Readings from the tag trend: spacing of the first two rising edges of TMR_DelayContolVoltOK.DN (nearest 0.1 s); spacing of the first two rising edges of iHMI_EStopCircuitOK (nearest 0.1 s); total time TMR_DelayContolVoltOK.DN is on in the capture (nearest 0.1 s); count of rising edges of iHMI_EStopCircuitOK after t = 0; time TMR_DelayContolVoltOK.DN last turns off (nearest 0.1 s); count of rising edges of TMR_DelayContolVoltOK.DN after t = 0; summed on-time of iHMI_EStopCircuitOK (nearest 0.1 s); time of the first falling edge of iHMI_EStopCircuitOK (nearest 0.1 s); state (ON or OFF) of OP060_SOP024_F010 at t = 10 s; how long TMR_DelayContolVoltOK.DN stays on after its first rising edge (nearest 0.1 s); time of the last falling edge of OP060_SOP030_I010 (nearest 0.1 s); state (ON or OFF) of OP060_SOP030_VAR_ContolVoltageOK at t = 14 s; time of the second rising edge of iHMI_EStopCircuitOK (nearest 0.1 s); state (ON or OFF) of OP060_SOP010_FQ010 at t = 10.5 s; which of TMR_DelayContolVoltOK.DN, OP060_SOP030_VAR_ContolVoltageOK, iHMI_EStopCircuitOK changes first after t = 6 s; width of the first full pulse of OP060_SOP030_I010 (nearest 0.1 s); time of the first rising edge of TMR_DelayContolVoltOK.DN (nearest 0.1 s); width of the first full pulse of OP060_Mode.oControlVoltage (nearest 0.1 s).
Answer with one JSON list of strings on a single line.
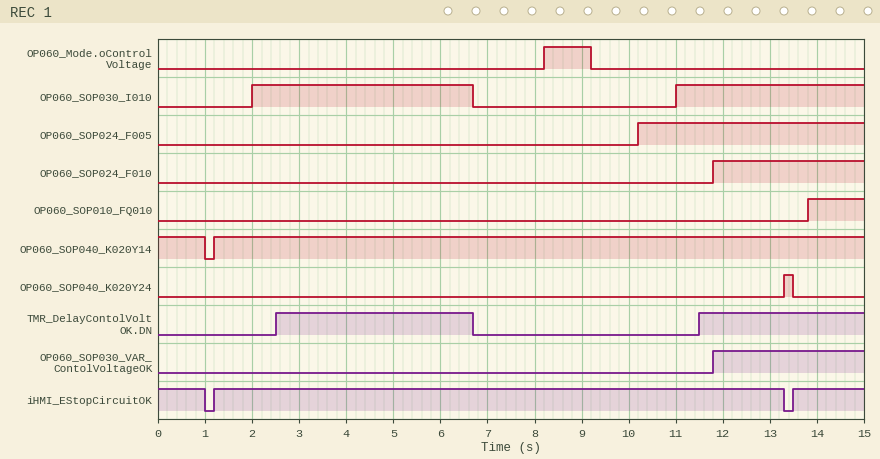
["9.0 s", "12.3 s", "7.7 s", "2", "6.7 s", "2", "14.6 s", "1.0 s", "OFF", "4.2 s", "6.7 s", "ON", "13.5 s", "OFF", "TMR_DelayContolVoltOK.DN", "4.7 s", "2.5 s", "1.0 s"]
